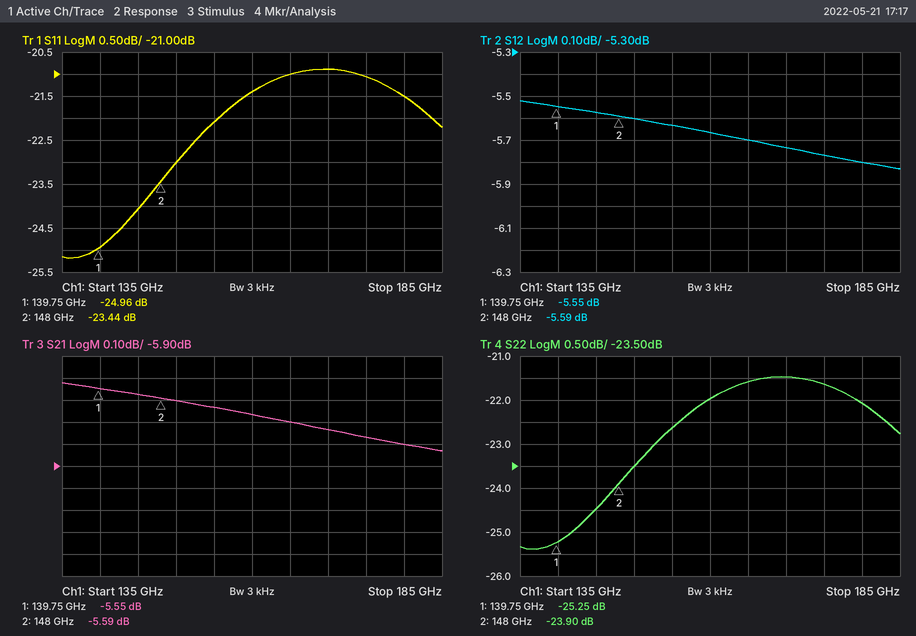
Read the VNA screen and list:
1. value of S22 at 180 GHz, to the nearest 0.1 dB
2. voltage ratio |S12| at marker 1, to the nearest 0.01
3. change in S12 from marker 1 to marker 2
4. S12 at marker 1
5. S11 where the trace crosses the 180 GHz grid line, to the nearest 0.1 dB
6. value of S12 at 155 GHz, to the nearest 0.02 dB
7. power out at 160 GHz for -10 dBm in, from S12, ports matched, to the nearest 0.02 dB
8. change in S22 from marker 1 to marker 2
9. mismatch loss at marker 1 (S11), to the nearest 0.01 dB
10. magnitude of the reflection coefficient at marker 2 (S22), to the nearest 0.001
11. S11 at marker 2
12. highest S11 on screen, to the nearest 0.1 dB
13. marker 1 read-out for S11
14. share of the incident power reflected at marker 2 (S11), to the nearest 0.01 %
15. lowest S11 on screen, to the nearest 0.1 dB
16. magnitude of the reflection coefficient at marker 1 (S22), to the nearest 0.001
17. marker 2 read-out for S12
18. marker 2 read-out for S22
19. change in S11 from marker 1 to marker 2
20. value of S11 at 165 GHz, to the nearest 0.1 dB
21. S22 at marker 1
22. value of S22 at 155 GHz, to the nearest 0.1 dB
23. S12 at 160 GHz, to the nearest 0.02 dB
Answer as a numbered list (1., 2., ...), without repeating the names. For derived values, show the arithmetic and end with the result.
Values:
1. -22.1 dB
2. 10^(-5.55/20) ≈ 0.53
3. -5.59 − (-5.55) = -0.04 dB
4. -5.55 dB
5. -21.5 dB
6. -5.64 dB
7. -10 dBm + (-5.66 dB) = -15.66 dBm
8. -23.9 − (-25.25) = 1.35 dB
9. −10 log10(1 − 10^(-24.96/10)) ≈ 0.01 dB
10. 10^(-23.9/20) ≈ 0.064
11. -23.44 dB
12. -20.9 dB
13. -24.96 dB
14. 10^(-23.44/10) ≈ 0.45 %
15. -25.2 dB
16. 10^(-25.25/20) ≈ 0.055
17. -5.59 dB
18. -23.90 dB
19. -23.44 − (-24.96) = 1.52 dB
20. -21.0 dB
21. -25.25 dB
22. -22.6 dB
23. -5.66 dB
